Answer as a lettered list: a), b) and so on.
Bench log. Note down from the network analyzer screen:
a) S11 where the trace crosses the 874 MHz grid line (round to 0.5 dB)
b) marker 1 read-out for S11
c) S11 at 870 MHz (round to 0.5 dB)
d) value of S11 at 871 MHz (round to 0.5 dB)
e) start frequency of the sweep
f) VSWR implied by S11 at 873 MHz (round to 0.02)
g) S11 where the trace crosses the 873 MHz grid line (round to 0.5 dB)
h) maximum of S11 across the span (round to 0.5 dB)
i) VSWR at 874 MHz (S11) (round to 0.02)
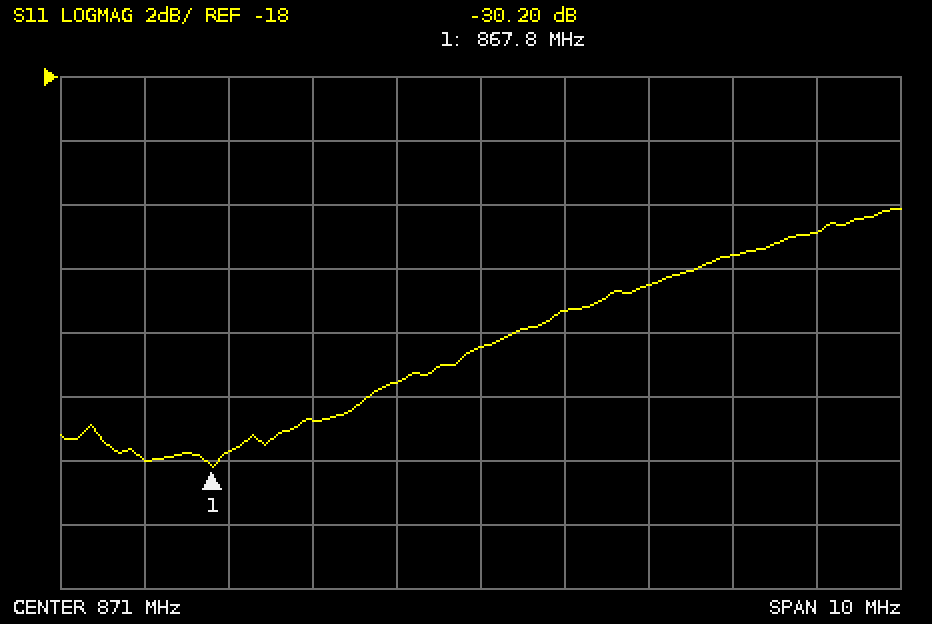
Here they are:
a) -23.5 dB
b) -30.20 dB
c) -27.5 dB
d) -26.5 dB
e) 866 MHz
f) 1.12
g) -24.5 dB
h) -22.0 dB
i) 1.14
